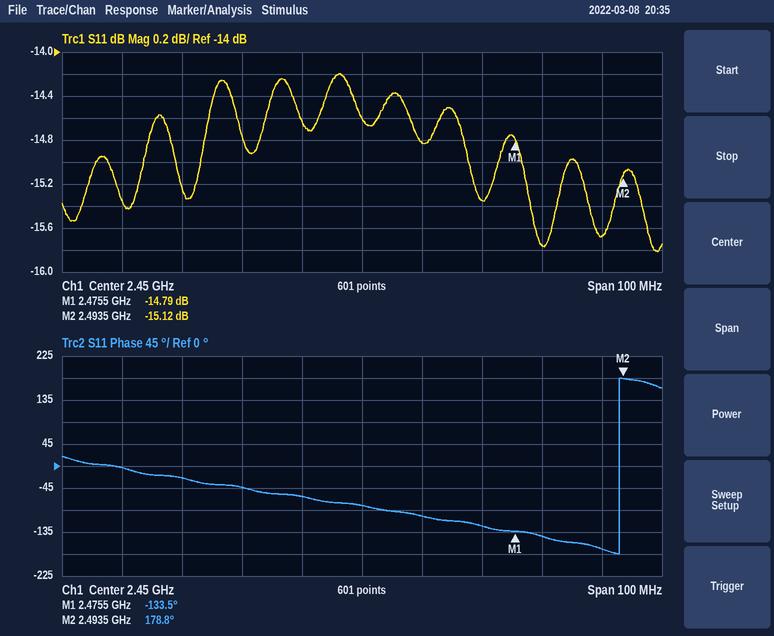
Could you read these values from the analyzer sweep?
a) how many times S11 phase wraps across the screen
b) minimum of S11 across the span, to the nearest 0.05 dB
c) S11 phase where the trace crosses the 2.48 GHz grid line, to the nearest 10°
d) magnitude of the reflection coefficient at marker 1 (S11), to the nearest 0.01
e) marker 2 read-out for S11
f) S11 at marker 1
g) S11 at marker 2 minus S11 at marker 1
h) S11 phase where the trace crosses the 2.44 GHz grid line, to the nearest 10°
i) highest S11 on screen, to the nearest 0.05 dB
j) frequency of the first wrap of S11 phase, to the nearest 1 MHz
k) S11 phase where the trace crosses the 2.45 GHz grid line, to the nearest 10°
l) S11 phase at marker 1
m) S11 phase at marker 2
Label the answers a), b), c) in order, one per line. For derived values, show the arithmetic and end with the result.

a) 1
b) -15.80 dB
c) -140°
d) 10^(-14.79/20) ≈ 0.18
e) -15.12 dB
f) -14.79 dB
g) -15.12 − (-14.79) = -0.33 dB
h) -60°
i) -14.20 dB
j) 2.493 GHz
k) -80°
l) -133.5°
m) 178.8°
